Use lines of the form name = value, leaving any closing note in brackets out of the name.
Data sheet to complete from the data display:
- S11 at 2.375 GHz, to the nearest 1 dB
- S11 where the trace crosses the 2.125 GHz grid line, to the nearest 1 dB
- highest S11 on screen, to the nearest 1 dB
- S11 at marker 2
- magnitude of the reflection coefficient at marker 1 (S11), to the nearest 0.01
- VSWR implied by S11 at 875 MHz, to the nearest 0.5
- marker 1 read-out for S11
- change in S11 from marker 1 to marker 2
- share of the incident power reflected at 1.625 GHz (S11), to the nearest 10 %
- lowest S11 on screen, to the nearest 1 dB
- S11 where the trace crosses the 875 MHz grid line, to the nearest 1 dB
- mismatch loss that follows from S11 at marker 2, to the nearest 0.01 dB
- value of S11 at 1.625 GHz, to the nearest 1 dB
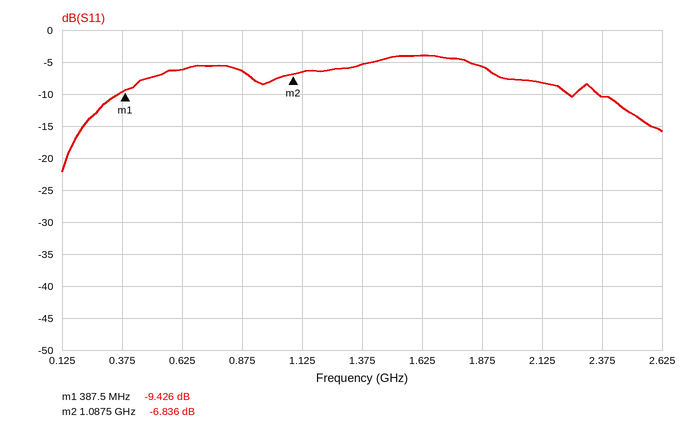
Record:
S11 at 2.375 GHz, to the nearest 1 dB = -10 dB
S11 where the trace crosses the 2.125 GHz grid line, to the nearest 1 dB = -8 dB
highest S11 on screen, to the nearest 1 dB = -4 dB
S11 at marker 2 = -6.836 dB
magnitude of the reflection coefficient at marker 1 (S11), to the nearest 0.01 = 0.34
VSWR implied by S11 at 875 MHz, to the nearest 0.5 = 3.0
marker 1 read-out for S11 = -9.426 dB
change in S11 from marker 1 to marker 2 = 2.590 dB
share of the incident power reflected at 1.625 GHz (S11), to the nearest 10 % = 40 %
lowest S11 on screen, to the nearest 1 dB = -22 dB
S11 where the trace crosses the 875 MHz grid line, to the nearest 1 dB = -6 dB
mismatch loss that follows from S11 at marker 2, to the nearest 0.01 dB = 1.01 dB
value of S11 at 1.625 GHz, to the nearest 1 dB = -4 dB
